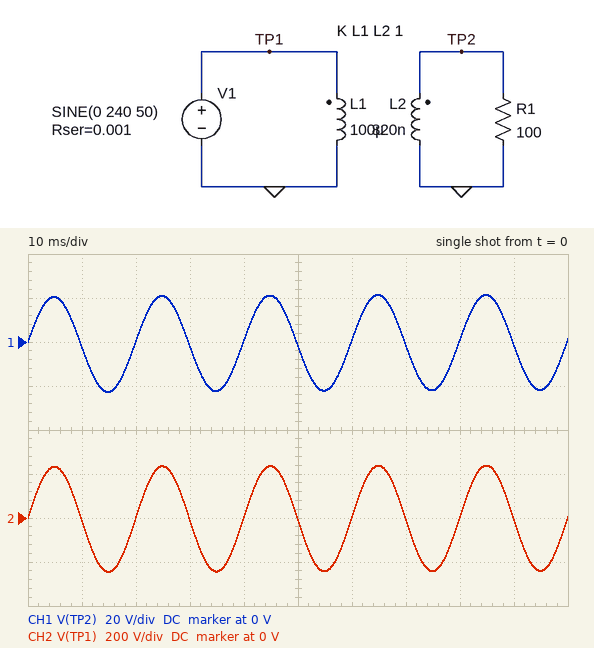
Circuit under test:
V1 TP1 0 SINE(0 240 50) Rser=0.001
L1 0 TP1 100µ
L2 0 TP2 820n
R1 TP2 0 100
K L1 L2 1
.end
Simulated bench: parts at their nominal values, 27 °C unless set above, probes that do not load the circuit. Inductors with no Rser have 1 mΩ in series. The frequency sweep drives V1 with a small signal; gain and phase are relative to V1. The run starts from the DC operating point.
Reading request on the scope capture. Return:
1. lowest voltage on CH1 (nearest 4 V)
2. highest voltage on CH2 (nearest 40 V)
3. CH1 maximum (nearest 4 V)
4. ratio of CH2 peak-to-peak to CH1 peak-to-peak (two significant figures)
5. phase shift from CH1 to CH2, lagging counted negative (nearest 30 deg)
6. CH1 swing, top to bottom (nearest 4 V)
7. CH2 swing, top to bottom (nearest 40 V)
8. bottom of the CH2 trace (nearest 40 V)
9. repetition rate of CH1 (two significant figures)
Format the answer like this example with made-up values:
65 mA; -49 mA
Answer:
-24 V; 240 V; 20 V; 11; 0 deg; 44 V; 480 V; -240 V; 50 Hz
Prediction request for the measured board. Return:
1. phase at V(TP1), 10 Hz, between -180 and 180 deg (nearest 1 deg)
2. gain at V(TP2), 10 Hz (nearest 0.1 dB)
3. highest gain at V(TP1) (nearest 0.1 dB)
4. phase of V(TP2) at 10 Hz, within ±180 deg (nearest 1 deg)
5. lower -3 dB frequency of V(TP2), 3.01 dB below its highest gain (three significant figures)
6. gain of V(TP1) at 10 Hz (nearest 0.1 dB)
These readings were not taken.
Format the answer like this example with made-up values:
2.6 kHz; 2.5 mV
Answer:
9 deg; -21.3 dB; 0 dB; 18 deg; 3.18 Hz; -0.3 dB
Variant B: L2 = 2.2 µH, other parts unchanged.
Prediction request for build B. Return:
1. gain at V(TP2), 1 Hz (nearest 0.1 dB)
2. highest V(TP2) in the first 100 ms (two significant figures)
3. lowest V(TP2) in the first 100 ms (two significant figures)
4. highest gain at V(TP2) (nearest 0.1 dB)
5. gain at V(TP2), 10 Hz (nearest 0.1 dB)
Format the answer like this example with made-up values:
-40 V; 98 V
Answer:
-27.0 dB; 35 V; -37 V; -16.6 dB; -17.0 dB
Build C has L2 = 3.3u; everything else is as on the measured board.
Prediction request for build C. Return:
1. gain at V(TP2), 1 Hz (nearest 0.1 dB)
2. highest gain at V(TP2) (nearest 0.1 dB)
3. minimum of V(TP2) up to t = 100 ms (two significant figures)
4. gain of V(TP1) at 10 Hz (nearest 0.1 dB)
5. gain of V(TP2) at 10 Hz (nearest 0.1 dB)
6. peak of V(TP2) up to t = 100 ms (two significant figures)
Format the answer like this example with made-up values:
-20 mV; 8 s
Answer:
-25.3 dB; -14.8 dB; -46 V; -0.3 dB; -15.2 dB; 43 V
